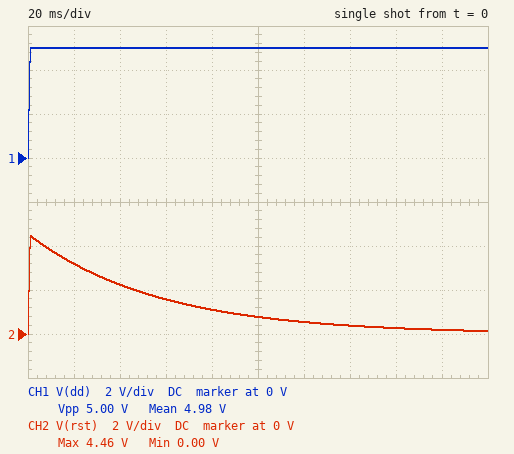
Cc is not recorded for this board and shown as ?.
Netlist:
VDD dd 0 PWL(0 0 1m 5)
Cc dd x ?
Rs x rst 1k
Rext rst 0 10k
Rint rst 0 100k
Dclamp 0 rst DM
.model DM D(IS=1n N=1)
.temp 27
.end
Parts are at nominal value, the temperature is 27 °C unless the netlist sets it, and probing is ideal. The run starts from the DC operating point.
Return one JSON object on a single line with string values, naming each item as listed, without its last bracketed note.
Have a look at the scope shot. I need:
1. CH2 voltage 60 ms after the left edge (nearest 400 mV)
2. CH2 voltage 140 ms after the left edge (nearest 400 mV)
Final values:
{"CH2 voltage 60 ms after the left edge": "1.6 V", "CH2 voltage 140 ms after the left edge": "400 mV"}
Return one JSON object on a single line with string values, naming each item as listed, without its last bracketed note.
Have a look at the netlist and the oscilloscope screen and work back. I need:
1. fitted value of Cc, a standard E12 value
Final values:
{"fitted value of Cc, a standard E12 value": "5.6 µF"}
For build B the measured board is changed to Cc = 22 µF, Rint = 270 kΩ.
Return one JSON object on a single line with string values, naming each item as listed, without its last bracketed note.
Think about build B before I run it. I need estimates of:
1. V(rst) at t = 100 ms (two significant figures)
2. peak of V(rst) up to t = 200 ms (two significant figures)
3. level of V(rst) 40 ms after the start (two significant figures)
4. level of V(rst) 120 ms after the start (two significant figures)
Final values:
{"V(rst) at t = 100 ms": "3.0 V", "peak of V(rst) up to t = 200 ms": "4.5 V", "level of V(rst) 40 ms after the start": "3.8 V", "level of V(rst) 120 ms after the start": "2.7 V"}
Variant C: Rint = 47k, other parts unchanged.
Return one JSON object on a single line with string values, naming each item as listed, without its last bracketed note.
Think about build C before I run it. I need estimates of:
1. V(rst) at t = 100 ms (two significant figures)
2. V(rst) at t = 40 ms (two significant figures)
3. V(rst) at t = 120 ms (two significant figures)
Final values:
{"V(rst) at t = 100 ms": "650 mV", "V(rst) at t = 40 ms": "2.1 V", "V(rst) at t = 120 ms": "440 mV"}
